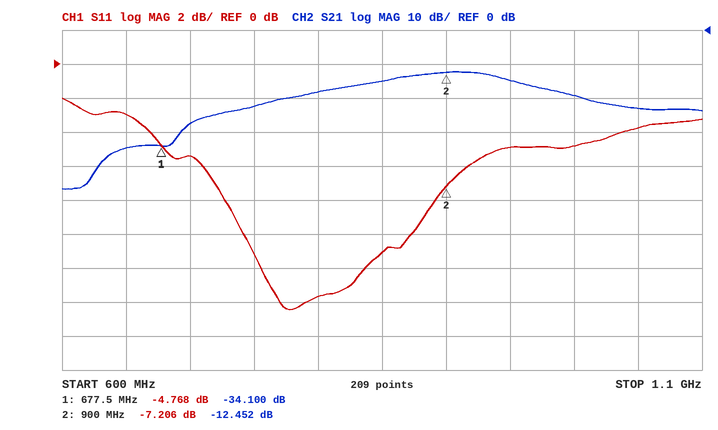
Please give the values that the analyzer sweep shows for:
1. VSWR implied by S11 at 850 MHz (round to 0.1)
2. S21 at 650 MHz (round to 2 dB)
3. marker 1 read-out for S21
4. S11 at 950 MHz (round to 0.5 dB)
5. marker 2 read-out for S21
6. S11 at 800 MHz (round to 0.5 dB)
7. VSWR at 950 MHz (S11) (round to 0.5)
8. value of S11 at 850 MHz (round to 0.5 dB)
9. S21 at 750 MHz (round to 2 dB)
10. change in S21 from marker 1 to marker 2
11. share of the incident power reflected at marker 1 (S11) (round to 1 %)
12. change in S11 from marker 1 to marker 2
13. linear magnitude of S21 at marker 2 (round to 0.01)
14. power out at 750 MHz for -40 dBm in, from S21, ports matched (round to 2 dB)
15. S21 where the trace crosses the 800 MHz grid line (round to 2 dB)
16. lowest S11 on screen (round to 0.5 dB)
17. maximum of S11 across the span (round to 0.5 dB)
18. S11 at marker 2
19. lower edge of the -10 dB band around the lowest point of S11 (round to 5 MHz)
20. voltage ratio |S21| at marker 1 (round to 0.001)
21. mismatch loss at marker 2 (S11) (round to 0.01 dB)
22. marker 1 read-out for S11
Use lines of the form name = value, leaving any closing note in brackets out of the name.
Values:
VSWR implied by S11 at 850 MHz = 1.8
S21 at 650 MHz = -34 dB
marker 1 read-out for S21 = -34.100 dB
S11 at 950 MHz = -5.0 dB
marker 2 read-out for S21 = -12.452 dB
S11 at 800 MHz = -13.5 dB
VSWR at 950 MHz (S11) = 3.5
value of S11 at 850 MHz = -11.0 dB
S21 at 750 MHz = -22 dB
change in S21 from marker 1 to marker 2 = 21.648 dB
share of the incident power reflected at marker 1 (S11) = 33 %
change in S11 from marker 1 to marker 2 = -2.438 dB
linear magnitude of S21 at marker 2 = 0.24
power out at 750 MHz for -40 dBm in, from S21, ports matched = -62 dBm
S21 where the trace crosses the 800 MHz grid line = -18 dB
lowest S11 on screen = -14.5 dB
maximum of S11 across the span = -2.0 dB
S11 at marker 2 = -7.206 dB
lower edge of the -10 dB band around the lowest point of S11 = 740 MHz
voltage ratio |S21| at marker 1 = 0.020
mismatch loss at marker 2 (S11) = 0.92 dB
marker 1 read-out for S11 = -4.768 dB
